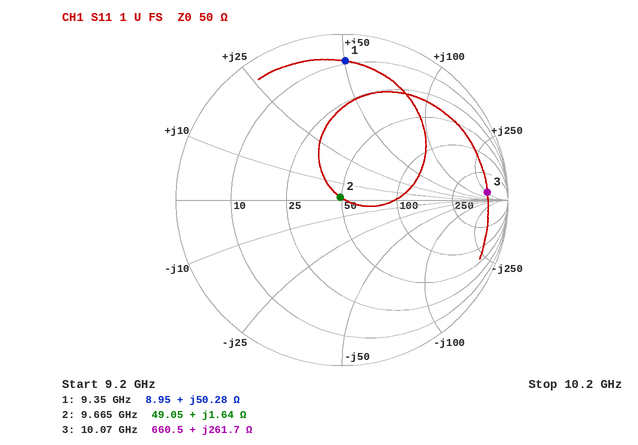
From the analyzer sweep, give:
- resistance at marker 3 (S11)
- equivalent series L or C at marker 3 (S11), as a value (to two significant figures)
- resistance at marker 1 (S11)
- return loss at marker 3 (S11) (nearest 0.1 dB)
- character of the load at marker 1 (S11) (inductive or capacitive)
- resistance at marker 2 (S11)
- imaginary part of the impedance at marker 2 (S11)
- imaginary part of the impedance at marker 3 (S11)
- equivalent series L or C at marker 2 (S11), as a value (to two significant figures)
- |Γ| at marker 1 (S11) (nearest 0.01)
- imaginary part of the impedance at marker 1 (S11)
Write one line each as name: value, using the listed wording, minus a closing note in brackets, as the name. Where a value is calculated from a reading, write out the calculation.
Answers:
resistance at marker 3: 660.5 Ω
equivalent series L or C at marker 3 (S11), as a value: L = 261.7 Ω/(2π × 10.07 GHz) ≈ 4.1 nH
resistance at marker 1: 8.95 Ω
return loss at marker 3 (S11): 1.1 dB
character of the load at marker 1 (S11): inductive
resistance at marker 2: 49.05 Ω
imaginary part of the impedance at marker 2: +1.64 Ω
imaginary part of the impedance at marker 3: +261.7 Ω
equivalent series L or C at marker 2 (S11), as a value: L = 1.64 Ω/(2π × 9.665 GHz) ≈ 27 pH
|Γ| at marker 1 (S11): 0.84
imaginary part of the impedance at marker 1: +50.28 Ω
